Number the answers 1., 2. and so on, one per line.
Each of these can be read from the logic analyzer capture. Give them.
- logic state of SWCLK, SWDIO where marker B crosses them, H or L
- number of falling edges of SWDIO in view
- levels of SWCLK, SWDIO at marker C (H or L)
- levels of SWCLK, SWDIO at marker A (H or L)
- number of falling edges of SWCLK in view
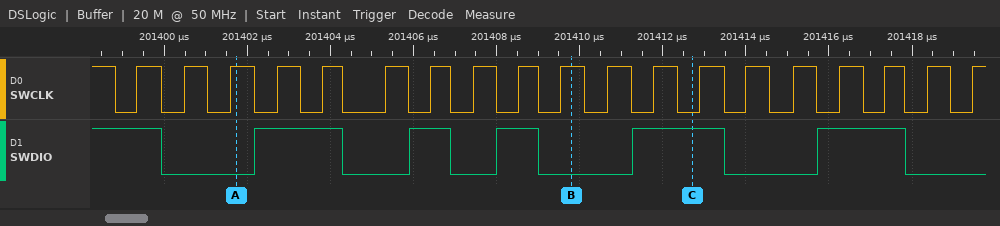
1. SWCLK=H, SWDIO=L
2. 6
3. SWCLK=L, SWDIO=H
4. SWCLK=H, SWDIO=L
5. 19
